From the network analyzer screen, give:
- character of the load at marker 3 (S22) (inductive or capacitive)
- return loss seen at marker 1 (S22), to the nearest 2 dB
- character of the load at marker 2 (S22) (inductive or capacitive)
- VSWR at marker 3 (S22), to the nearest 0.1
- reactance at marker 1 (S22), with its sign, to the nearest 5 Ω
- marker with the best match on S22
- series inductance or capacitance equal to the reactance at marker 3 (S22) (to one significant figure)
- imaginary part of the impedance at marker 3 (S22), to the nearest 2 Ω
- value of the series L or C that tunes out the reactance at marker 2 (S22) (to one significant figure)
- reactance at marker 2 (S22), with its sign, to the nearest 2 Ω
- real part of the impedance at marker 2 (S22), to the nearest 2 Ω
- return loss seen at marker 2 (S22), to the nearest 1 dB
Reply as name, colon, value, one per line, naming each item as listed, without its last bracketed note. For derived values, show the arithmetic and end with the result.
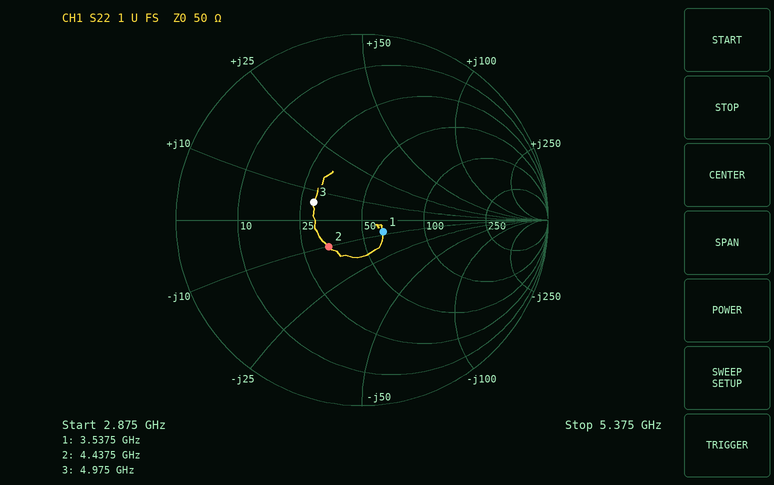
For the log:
character of the load at marker 3 (S22): inductive
return loss seen at marker 1 (S22), to the nearest 2 dB: 18 dB
character of the load at marker 2 (S22): capacitive
VSWR at marker 3 (S22), to the nearest 0.1: 1.8
reactance at marker 1 (S22), with its sign, to the nearest 5 Ω: -10 Ω
marker with the best match on S22: marker 1
series inductance or capacitance equal to the reactance at marker 3 (S22): L = 6 Ω/(2π × 4.975 GHz) ≈ 192 pH, so 200 pH to one significant figure
imaginary part of the impedance at marker 3 (S22), to the nearest 2 Ω: +6 Ω
value of the series L or C that tunes out the reactance at marker 2 (S22): L = 10 Ω/(2π × 4.4375 GHz) ≈ 359 pH, so 400 pH to one significant figure
reactance at marker 2 (S22), with its sign, to the nearest 2 Ω: -10 Ω
real part of the impedance at marker 2 (S22), to the nearest 2 Ω: 34 Ω
return loss seen at marker 2 (S22), to the nearest 1 dB: 13 dB
